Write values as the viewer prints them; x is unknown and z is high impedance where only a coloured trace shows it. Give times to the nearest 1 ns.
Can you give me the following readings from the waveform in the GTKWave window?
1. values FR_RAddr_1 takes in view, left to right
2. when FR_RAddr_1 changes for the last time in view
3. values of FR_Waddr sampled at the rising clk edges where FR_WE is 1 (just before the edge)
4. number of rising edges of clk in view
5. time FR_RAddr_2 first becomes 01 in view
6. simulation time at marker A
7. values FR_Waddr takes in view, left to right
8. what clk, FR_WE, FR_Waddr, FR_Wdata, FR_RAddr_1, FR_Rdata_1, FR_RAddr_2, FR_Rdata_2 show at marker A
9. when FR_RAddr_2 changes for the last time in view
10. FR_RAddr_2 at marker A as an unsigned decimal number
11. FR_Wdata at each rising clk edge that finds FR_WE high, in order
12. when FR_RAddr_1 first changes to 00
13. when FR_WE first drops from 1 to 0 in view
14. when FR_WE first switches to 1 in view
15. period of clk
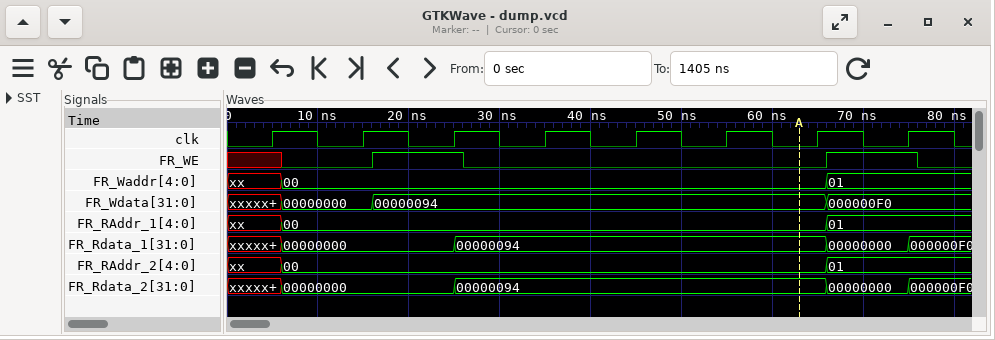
xx, 00, 01
66 ns
00, 01
8
66 ns
63 ns
xx, 00, 01
clk=0, FR_WE=0, FR_Waddr=00, FR_Wdata=00000094, FR_RAddr_1=00, FR_Rdata_1=00000094, FR_RAddr_2=00, FR_Rdata_2=00000094
66 ns
0
00000094, 000000F0
6 ns
26 ns
16 ns
10 ns
